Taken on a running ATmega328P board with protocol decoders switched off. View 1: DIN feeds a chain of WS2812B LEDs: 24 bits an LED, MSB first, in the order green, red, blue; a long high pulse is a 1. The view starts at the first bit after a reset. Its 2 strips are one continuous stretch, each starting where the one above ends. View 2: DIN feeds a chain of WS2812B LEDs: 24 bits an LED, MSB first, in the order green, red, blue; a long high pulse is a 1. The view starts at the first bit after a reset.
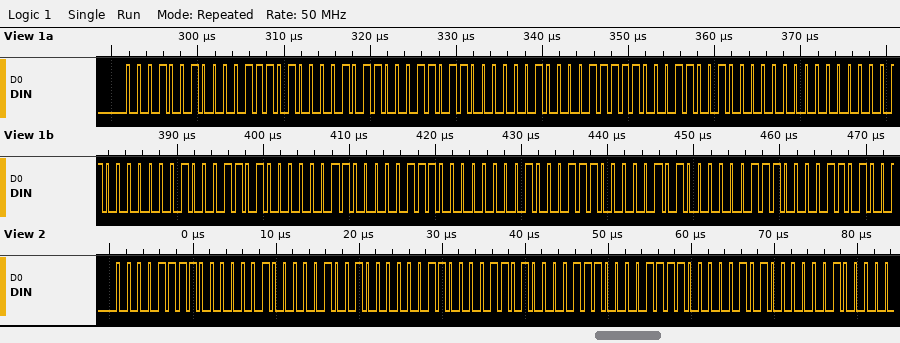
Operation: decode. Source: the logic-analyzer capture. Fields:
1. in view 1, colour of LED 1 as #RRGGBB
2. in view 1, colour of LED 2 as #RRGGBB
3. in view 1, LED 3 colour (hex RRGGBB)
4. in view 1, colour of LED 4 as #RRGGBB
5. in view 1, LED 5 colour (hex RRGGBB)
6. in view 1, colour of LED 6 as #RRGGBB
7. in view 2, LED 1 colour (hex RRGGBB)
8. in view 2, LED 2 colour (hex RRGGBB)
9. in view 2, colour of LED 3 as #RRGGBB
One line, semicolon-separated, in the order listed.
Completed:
#1D120B; #021B1F; #001901; #1A0106; #010E1C; #0E141A; #020F09; #0D030E; #0A1E04
